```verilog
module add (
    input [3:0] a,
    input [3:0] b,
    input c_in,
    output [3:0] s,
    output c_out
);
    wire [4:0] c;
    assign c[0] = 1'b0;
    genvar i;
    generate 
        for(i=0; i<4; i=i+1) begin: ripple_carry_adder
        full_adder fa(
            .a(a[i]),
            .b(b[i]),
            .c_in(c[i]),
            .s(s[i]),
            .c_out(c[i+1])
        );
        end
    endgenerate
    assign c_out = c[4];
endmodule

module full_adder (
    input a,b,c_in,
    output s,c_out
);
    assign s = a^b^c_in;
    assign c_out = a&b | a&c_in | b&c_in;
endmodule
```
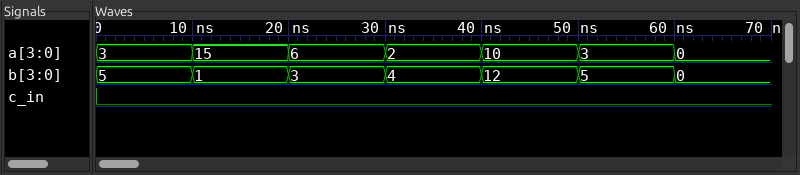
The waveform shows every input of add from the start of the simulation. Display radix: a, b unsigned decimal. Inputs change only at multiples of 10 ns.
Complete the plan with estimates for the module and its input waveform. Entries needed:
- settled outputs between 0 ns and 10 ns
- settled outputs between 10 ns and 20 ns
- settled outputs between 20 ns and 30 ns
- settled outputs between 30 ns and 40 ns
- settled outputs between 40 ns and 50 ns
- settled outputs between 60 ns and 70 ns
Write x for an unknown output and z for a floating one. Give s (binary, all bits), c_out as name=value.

s=1000, c_out=0
s=0000, c_out=1
s=1001, c_out=0
s=0110, c_out=0
s=0110, c_out=1
s=0000, c_out=0
